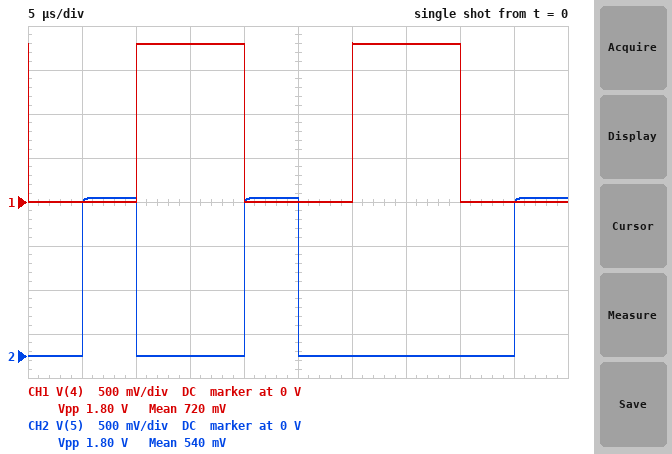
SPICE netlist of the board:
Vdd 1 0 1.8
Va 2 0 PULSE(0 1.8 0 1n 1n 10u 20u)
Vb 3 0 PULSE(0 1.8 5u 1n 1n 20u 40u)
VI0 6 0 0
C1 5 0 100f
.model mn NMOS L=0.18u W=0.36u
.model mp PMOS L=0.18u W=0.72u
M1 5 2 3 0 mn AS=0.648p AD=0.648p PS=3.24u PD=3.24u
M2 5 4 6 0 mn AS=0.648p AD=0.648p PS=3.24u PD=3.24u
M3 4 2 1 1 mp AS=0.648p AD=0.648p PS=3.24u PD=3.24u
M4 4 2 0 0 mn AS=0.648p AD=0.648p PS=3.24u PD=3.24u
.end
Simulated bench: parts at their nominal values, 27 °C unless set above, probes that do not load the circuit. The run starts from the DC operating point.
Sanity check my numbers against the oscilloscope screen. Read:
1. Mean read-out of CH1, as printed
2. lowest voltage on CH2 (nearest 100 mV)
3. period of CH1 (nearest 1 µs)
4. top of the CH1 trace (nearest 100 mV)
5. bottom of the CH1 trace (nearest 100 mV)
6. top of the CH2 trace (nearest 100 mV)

720 mV
0 V
20 µs
1.8 V
0 V
1.8 V
